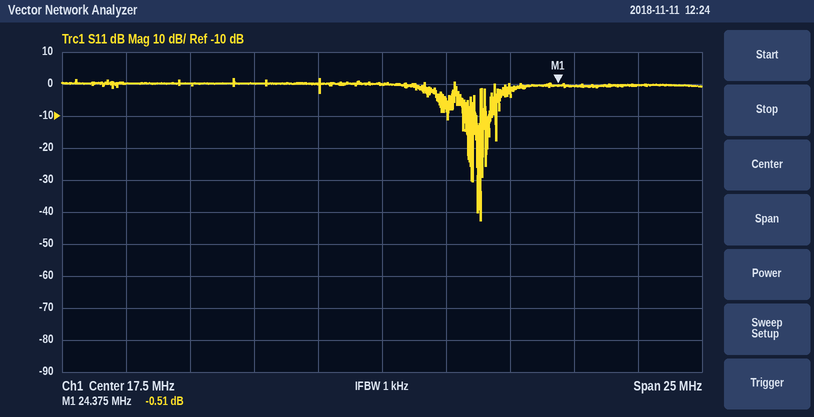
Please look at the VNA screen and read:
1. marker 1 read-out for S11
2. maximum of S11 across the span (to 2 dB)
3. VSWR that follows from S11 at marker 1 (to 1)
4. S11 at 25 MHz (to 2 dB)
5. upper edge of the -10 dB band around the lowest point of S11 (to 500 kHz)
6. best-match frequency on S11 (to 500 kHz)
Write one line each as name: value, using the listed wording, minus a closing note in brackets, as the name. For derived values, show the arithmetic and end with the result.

marker 1 read-out for S11: -0.51 dB
maximum of S11 across the span: 2 dB
VSWR that follows from S11 at marker 1: (1 + 0.9430)/(1 − 0.9430) ≈ 34
S11 at 25 MHz: 0 dB
upper edge of the -10 dB band around the lowest point of S11: 21.5 MHz
best-match frequency on S11: 21.5 MHz
